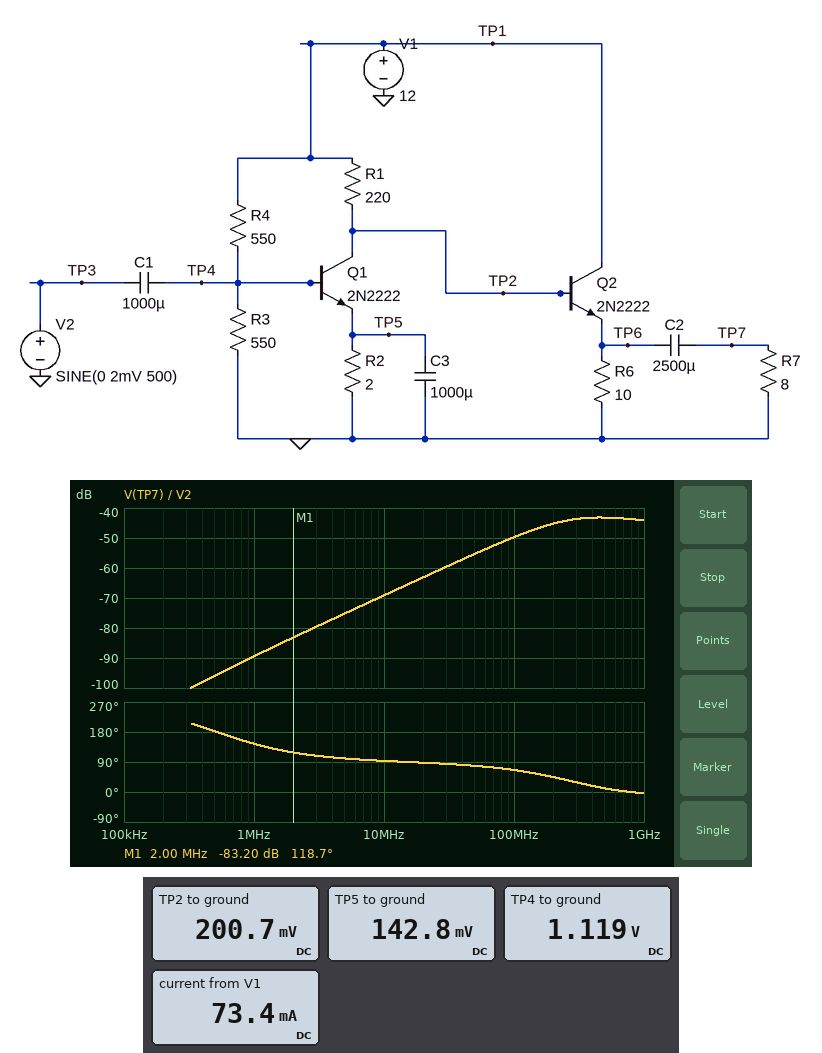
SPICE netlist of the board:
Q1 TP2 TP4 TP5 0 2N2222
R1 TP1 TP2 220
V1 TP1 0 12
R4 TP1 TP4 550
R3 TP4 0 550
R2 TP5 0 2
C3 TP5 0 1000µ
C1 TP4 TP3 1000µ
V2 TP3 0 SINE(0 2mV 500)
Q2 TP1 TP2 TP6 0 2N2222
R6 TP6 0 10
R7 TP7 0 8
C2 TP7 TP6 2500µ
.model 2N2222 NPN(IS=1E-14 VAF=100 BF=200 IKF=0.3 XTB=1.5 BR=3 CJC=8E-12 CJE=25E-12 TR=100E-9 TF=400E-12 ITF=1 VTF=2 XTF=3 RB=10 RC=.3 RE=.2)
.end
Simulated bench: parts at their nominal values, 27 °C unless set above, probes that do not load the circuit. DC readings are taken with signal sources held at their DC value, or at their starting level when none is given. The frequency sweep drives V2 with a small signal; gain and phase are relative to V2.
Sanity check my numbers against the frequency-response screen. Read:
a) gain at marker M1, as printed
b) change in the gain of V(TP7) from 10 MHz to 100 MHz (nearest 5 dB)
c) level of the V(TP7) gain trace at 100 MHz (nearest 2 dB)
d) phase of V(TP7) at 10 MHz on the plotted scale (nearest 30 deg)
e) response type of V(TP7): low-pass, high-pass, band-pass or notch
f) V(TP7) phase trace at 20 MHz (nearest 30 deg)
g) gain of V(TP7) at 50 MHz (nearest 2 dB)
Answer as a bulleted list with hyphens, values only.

- -83.20 dB
- 20 dB
- -50 dB
- 90 deg
- high-pass
- 90 deg
- -56 dB
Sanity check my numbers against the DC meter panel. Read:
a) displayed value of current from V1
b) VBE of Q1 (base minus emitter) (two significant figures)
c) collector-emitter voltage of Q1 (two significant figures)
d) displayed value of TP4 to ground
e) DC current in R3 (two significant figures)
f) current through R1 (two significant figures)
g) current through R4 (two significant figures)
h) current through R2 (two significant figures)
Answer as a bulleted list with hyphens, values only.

- 73.4 mA
- 980 mV
- 58 mV
- 1.119 V
- 2.0 mA
- 54 mA
- 20 mA
- 71 mA
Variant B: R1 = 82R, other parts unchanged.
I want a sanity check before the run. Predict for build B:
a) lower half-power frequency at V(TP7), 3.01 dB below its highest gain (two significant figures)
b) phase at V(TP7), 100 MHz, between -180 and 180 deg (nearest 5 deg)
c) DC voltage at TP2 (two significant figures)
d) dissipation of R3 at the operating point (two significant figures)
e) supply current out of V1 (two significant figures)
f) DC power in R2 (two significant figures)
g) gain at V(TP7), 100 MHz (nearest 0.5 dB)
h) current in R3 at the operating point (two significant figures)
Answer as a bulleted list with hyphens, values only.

- 150 MHz
- 65 deg
- 440 mV
- 3.2 mW
- 160 mA
- 50 mW
- -50.5 dB
- 2.4 mA
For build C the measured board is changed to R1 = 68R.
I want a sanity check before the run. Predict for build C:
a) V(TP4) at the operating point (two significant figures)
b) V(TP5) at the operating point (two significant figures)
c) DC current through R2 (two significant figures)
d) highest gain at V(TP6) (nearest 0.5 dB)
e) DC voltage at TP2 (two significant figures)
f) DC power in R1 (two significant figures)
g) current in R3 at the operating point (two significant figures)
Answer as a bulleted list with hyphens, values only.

- 1.4 V
- 370 mV
- 190 mA
- -45.0 dB
- 510 mV
- 1.9 W
- 2.5 mA
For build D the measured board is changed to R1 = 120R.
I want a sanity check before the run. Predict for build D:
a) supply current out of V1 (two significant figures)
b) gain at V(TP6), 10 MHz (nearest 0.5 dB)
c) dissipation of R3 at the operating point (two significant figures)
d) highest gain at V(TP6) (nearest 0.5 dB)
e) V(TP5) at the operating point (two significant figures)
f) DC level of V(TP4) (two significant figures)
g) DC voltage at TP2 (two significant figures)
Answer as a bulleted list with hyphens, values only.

- 120 mA
- -69.5 dB
- 2.7 mW
- -44.0 dB
- 230 mV
- 1.2 V
- 320 mV
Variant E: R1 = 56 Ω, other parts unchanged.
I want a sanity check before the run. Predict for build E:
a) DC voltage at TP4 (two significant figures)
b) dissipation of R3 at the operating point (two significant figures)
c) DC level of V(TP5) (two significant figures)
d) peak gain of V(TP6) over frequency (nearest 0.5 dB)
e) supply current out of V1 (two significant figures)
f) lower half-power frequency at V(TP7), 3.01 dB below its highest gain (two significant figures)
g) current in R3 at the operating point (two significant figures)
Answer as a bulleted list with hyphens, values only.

- 1.5 V
- 3.9 mW
- 440 mV
- -45.0 dB
- 220 mA
- 130 MHz
- 2.7 mA
